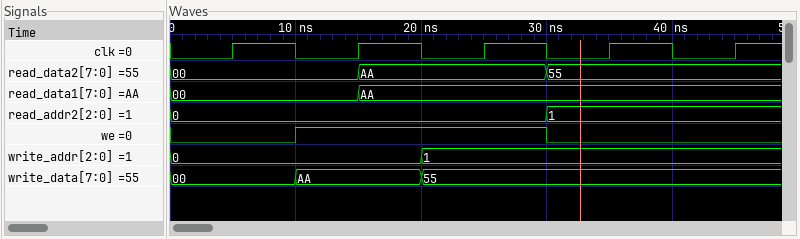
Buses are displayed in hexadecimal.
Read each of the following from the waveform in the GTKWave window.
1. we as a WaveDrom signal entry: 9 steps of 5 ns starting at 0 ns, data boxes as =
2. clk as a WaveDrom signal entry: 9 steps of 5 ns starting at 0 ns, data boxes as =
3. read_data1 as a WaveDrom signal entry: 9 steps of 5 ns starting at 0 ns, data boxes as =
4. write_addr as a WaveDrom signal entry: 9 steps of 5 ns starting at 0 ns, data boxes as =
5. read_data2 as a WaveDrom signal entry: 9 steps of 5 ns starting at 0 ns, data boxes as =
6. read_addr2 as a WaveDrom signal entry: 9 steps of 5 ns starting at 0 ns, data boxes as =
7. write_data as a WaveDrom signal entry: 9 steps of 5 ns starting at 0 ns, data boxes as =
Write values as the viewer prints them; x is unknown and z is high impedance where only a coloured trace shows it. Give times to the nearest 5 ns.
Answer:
{name: 'we', wave: '0.1...0..'}
{name: 'clk', wave: '010101010'}
{name: 'read_data1', wave: '=..=.....', data: '00 AA'}
{name: 'write_addr', wave: '=...=....', data: '0 1'}
{name: 'read_data2', wave: '=..=..=..', data: '00 AA 55'}
{name: 'read_addr2', wave: '=.....=..', data: '0 1'}
{name: 'write_data', wave: '=.=.=....', data: '00 AA 55'}
